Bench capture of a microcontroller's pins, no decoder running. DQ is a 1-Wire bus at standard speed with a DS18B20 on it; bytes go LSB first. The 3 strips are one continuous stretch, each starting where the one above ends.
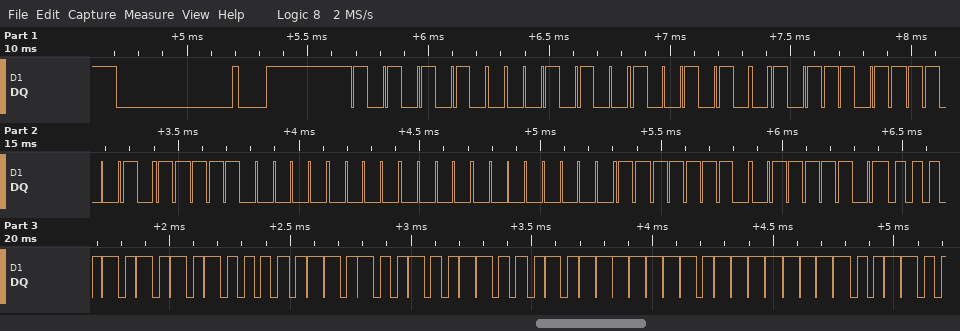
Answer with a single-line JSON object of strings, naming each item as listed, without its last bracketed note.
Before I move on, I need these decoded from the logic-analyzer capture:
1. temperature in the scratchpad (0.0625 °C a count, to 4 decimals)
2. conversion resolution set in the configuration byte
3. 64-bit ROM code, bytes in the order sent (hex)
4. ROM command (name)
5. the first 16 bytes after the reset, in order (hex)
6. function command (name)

{"temperature in the scratchpad": "85.0000 °C", "conversion resolution set in the configuration byte": "12 bits", "64-bit ROM code, bytes in the order sent": "28 29 DD D3 07 00 00 7F", "ROM command": "Match ROM", "the first 16 bytes after the reset, in order": "55 28 29 DD D3 07 00 00 7F BE 50 05 4B 46 7F FF", "function command": "Read Scratchpad"}
